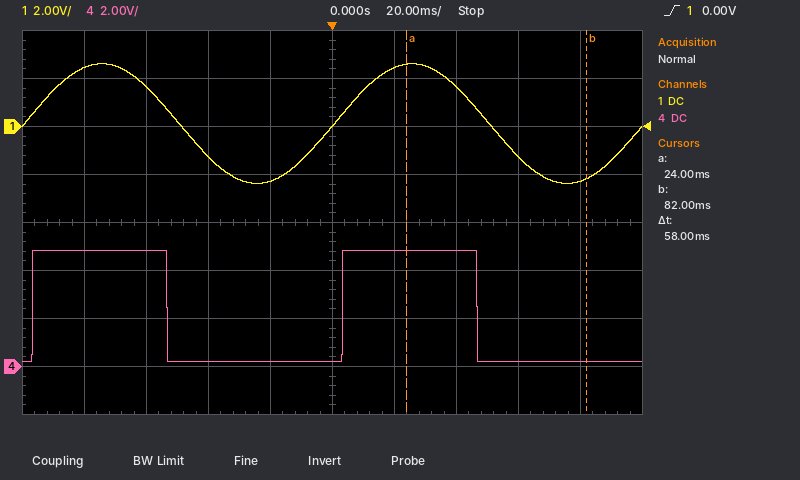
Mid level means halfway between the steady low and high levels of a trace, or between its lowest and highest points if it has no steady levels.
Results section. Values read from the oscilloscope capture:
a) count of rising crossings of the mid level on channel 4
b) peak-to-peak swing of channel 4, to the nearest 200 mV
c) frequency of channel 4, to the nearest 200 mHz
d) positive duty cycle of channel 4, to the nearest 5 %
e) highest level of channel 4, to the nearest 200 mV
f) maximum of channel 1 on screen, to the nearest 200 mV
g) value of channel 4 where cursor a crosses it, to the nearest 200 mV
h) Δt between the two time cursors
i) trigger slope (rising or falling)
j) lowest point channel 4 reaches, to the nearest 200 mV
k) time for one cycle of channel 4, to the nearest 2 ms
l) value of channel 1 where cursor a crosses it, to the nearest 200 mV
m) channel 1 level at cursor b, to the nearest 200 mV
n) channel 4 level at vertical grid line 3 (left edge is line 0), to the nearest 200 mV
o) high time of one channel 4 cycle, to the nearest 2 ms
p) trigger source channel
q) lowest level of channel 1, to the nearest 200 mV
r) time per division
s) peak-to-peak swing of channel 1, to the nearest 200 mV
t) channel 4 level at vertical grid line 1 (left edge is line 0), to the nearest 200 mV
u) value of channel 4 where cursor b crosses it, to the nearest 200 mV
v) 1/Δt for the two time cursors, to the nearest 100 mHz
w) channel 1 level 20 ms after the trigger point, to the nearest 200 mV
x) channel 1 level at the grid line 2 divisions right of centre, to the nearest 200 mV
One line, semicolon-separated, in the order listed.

2; 4.6 V; 10.0 Hz; 45 %; 4.8 V; 2.6 V; 4.8 V; 58 ms; rising; 200 mV; 100 ms; 2.6 V; -2.2 V; 200 mV; 44 ms; channel 1; -2.4 V; 20 ms; 5.0 V; 4.8 V; 200 mV; 17.2 Hz; 2.4 V; 1.6 V
